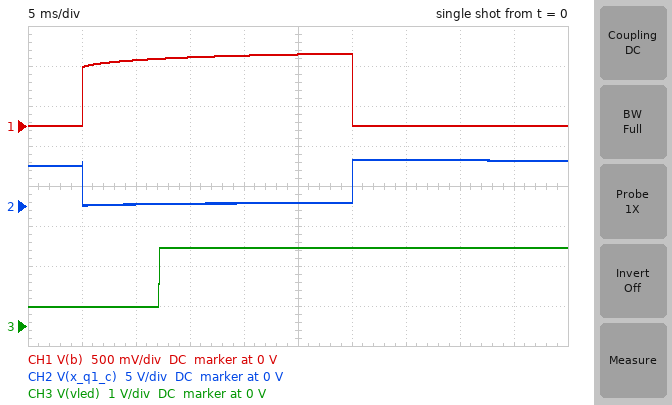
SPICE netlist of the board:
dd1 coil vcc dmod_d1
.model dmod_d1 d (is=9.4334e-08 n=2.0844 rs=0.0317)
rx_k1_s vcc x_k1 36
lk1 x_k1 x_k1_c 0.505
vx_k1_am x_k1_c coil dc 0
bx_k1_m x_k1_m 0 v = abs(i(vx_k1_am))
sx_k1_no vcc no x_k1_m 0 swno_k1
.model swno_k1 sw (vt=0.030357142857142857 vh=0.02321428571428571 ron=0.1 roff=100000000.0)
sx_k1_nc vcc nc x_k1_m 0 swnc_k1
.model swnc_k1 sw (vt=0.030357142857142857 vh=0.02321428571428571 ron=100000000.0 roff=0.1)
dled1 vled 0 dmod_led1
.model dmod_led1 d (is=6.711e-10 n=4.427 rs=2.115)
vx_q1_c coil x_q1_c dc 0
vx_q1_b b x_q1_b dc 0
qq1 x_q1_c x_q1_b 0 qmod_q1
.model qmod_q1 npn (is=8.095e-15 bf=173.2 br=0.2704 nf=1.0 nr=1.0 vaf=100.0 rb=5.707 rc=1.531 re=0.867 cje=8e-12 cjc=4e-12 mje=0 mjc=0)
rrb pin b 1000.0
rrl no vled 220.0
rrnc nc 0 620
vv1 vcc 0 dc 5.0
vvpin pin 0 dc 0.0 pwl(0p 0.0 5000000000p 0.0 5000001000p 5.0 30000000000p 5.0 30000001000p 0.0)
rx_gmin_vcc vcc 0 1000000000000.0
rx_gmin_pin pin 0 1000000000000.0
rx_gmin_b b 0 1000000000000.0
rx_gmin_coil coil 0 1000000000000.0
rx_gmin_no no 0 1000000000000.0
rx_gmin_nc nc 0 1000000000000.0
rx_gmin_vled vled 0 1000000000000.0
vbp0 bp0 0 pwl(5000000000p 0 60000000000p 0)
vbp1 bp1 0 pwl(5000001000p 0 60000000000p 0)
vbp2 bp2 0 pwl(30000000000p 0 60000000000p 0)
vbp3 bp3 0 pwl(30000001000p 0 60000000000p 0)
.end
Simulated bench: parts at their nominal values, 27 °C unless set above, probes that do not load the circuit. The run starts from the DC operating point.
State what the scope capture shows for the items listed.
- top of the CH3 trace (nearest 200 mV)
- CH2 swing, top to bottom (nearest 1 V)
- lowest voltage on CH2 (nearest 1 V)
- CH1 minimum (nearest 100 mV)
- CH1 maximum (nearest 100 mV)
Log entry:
2.0 V
6 V
0 V
0 V
900 mV
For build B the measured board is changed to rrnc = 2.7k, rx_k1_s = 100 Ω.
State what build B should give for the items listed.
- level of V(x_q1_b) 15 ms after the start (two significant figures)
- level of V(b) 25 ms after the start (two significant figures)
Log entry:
820 mV
830 mV
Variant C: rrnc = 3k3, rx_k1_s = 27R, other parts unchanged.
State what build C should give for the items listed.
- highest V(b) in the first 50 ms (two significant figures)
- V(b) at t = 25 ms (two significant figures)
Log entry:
920 mV
910 mV
